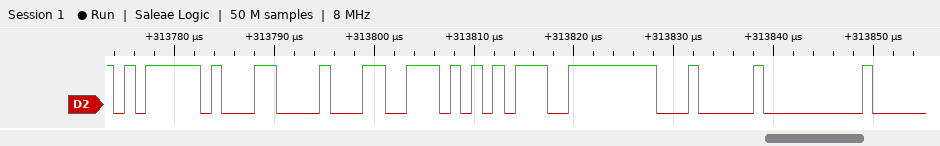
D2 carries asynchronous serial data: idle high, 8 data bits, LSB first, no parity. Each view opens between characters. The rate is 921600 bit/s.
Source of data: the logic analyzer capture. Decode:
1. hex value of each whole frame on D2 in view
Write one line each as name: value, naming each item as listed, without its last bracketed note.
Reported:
hex value of each whole frame on D2 in view: 7D, 0C, CC, D5, FE, 04, 00
